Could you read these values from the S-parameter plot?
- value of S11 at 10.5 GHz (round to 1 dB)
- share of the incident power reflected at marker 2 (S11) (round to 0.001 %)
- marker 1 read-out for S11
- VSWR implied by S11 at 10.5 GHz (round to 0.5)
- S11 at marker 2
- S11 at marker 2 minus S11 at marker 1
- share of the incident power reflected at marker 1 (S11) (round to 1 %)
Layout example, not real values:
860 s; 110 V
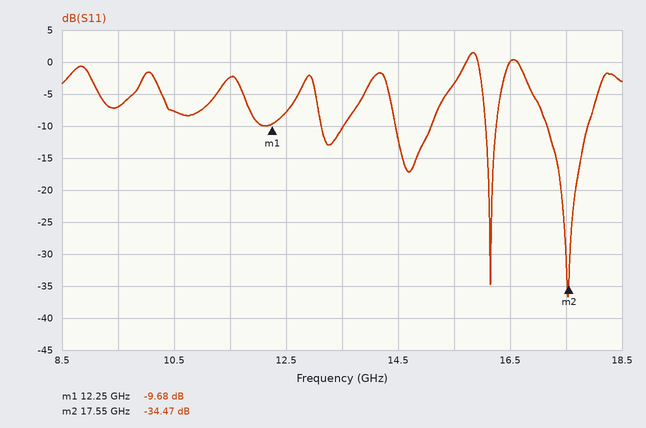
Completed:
-8 dB; 0.036 %; -9.68 dB; 2.5; -34.47 dB; -24.79 dB; 11 %
